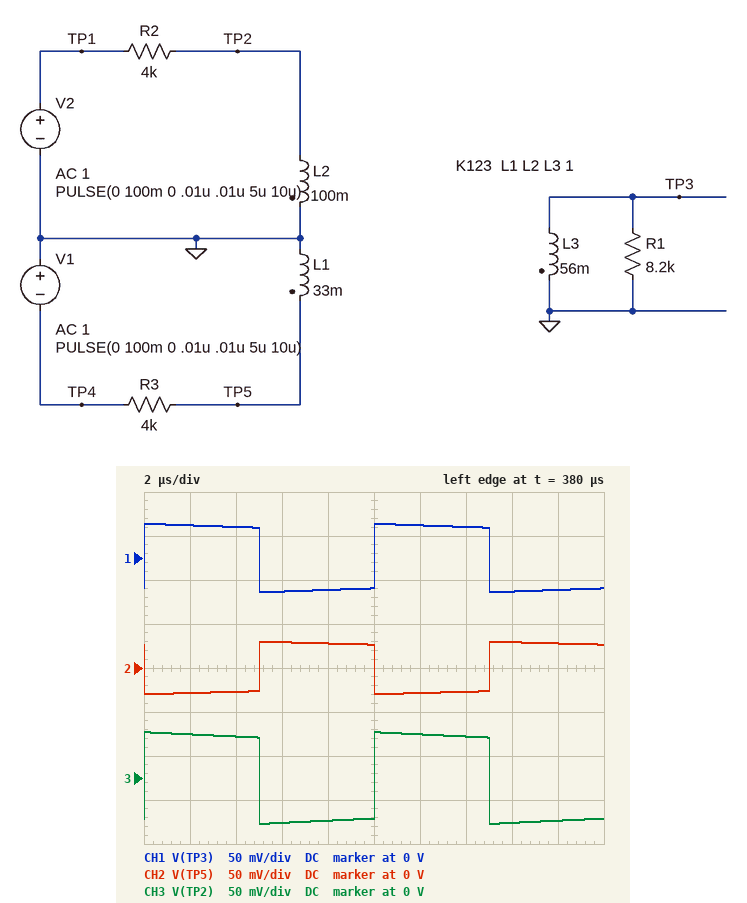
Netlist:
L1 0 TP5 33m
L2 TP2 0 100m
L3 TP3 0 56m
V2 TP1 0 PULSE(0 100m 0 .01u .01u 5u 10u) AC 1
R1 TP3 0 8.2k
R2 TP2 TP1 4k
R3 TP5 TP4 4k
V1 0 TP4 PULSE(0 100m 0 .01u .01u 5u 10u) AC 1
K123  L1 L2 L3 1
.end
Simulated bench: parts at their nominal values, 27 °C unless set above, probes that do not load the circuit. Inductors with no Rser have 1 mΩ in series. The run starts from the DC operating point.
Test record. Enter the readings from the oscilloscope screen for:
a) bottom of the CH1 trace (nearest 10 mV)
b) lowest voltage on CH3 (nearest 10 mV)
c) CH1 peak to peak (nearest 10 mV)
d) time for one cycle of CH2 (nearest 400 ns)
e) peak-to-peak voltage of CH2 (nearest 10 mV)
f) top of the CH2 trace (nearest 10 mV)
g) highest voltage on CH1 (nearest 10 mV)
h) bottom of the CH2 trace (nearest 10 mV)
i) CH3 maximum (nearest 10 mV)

-40 mV
-50 mV
80 mV
10.0 µs
60 mV
30 mV
40 mV
-30 mV
50 mV
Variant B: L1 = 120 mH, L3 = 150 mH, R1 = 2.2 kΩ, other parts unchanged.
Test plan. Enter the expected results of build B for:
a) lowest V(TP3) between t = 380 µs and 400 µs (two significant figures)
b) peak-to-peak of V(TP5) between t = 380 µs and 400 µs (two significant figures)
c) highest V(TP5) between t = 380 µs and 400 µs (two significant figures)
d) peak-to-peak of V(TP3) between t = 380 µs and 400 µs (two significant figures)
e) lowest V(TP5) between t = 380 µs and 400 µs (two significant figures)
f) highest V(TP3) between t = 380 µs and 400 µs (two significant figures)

-26 mV
48 mV
23 mV
53 mV
-25 mV
28 mV
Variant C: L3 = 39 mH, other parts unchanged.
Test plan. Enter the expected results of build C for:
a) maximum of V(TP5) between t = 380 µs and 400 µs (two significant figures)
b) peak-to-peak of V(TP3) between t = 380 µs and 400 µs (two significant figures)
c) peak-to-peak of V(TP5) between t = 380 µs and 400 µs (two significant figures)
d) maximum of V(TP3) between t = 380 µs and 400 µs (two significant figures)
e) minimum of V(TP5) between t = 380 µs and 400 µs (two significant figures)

32 mV
69 mV
63 mV
34 mV
-32 mV
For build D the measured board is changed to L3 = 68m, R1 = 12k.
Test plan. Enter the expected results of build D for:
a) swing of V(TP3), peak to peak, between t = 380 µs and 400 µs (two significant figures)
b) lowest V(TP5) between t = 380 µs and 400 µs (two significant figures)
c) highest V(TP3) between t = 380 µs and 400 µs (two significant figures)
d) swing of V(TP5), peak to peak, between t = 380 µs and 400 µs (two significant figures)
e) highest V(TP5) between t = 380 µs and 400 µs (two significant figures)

89 mV
-31 mV
44 mV
62 mV
31 mV
